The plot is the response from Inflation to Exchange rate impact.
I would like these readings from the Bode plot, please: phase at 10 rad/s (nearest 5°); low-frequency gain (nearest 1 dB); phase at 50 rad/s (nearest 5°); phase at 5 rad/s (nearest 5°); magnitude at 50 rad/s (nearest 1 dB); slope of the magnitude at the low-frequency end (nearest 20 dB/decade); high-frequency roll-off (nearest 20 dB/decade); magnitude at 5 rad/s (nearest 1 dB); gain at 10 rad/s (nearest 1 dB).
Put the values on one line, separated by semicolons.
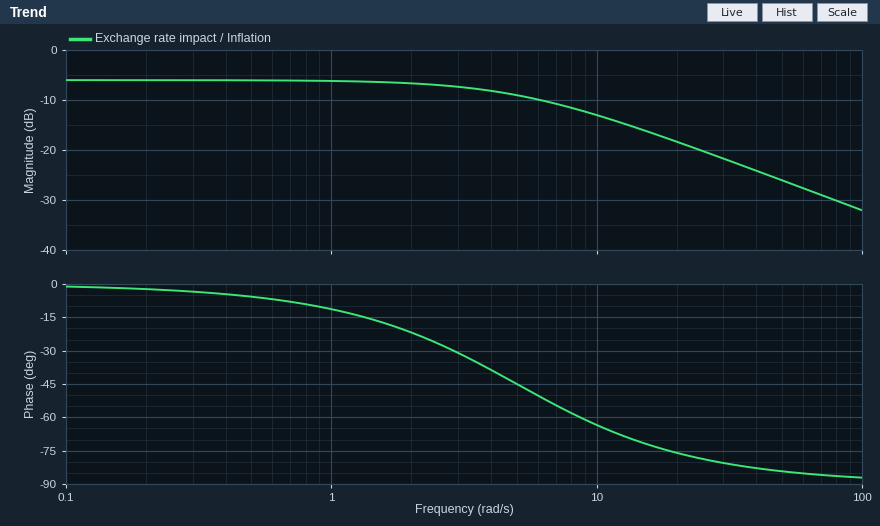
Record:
-65°; -6 dB; -85°; -45°; -26 dB; 0 dB/decade; -20 dB/decade; -9 dB; -13 dB
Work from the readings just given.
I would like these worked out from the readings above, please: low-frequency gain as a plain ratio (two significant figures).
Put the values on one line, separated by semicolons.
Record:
0.50
